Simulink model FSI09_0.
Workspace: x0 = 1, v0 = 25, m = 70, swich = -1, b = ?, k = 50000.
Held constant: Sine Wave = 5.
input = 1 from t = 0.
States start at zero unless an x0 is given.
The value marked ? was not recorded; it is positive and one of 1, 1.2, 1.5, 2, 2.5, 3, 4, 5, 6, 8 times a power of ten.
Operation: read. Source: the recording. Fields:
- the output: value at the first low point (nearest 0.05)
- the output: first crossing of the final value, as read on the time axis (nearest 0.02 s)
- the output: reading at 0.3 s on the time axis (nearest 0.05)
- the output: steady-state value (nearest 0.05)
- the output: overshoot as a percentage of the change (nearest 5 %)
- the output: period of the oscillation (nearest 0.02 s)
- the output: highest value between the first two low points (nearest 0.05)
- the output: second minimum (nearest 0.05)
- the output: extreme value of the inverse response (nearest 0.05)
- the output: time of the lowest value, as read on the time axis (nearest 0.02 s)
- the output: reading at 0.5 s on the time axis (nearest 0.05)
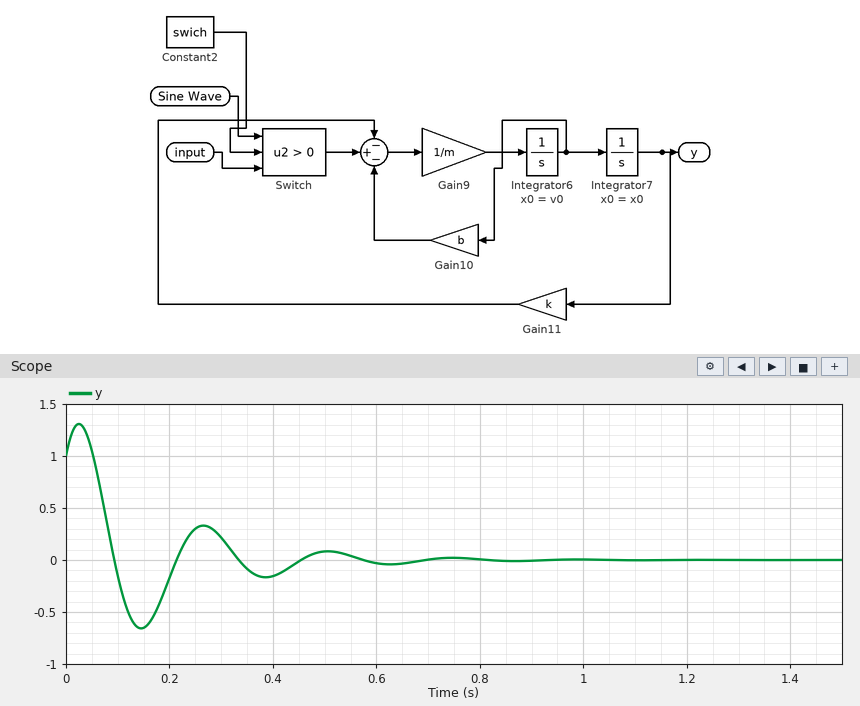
-0.65
0.10 s
0.20
0.00
65 %
0.24 s
0.35
-0.15
1.30
0.14 s
0.10
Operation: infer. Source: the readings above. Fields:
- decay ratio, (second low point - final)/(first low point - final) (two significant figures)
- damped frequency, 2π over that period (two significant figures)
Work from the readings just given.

0.23
26 rad/s
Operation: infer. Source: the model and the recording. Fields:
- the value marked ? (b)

800
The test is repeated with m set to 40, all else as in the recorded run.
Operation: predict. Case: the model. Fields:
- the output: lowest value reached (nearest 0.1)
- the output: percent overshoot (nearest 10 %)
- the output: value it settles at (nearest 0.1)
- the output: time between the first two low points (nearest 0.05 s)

-0.5
50 %
0.0
0.20 s
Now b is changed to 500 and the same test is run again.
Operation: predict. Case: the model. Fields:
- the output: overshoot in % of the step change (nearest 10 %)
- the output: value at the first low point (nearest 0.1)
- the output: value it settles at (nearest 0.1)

90 %
-0.9
0.0
